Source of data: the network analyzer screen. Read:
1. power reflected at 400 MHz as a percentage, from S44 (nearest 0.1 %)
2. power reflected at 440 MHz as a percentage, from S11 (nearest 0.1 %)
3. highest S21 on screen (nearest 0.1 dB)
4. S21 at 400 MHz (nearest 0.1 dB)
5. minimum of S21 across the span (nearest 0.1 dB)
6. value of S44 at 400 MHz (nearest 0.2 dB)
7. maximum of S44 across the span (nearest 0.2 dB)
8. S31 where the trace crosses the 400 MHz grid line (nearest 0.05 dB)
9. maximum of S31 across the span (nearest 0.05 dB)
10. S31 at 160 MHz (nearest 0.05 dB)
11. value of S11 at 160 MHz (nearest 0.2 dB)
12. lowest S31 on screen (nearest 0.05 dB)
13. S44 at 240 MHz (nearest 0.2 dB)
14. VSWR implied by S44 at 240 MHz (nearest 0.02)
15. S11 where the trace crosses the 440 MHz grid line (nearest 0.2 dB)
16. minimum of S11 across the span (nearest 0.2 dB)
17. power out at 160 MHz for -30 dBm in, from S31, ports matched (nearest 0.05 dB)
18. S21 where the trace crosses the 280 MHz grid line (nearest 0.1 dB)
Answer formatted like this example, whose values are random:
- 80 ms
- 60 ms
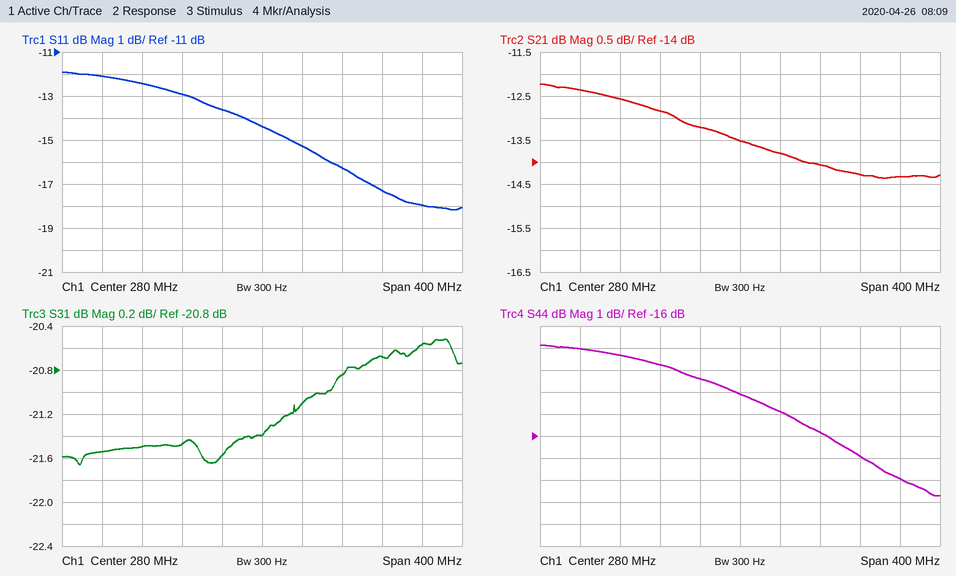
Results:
- 2.0 %
- 1.6 %
- -12.2 dB
- -14.3 dB
- -14.4 dB
- -17.0 dB
- -11.8 dB
- -20.70 dB
- -20.50 dB
- -21.50 dB
- -12.4 dB
- -21.65 dB
- -13.4 dB
- 1.54
- -18.0 dB
- -18.2 dB
- -51.50 dBm
- -13.5 dB
